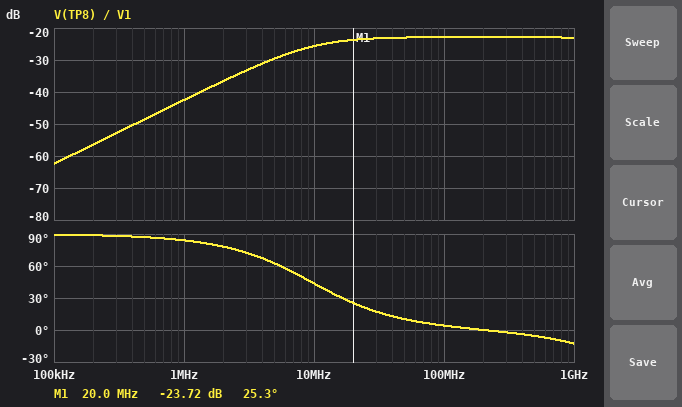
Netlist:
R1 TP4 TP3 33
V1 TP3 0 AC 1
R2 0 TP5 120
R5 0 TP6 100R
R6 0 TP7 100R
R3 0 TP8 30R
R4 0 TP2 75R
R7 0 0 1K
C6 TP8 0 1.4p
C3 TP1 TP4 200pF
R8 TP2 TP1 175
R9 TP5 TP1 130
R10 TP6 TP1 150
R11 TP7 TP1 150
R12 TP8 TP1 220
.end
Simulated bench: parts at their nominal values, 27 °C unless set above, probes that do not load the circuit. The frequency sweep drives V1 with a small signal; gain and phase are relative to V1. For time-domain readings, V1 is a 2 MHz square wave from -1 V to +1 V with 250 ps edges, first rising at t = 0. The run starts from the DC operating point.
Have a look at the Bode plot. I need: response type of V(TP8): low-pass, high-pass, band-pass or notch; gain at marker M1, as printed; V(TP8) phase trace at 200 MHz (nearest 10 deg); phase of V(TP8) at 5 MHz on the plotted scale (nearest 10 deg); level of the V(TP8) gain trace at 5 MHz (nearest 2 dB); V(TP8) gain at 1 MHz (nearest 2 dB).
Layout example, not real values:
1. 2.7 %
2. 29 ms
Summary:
1. high-pass
2. -23.72 dB
3. 0 deg
4. 60 deg
5. -30 dB
6. -42 dB
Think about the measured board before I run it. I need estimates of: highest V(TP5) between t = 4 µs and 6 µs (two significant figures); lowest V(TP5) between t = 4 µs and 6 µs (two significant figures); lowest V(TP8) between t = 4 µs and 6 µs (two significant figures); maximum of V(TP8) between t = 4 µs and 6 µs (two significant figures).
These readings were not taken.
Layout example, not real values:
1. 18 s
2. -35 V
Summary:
1. 570 mV
2. -570 mV
3. -140 mV
4. 140 mV
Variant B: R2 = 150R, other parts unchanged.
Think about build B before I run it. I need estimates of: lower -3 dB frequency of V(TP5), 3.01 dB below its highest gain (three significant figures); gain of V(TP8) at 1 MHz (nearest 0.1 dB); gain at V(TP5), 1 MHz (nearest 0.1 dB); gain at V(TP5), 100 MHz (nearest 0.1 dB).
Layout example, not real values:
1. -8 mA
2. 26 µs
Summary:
1. 9.46 MHz
2. -42.3 dB
3. -29.3 dB
4. -9.8 dB
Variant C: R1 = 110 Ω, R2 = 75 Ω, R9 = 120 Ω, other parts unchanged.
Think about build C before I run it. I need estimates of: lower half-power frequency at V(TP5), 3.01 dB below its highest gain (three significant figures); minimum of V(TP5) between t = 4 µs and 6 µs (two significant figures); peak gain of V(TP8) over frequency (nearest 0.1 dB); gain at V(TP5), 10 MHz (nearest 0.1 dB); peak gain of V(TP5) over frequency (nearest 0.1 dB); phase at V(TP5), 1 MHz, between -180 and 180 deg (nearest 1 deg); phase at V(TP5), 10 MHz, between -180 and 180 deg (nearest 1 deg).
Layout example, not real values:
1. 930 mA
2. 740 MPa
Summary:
1. 5.06 MHz
2. -230 mV
3. -28.9 dB
4. -19.7 dB
5. -18.7 dB
6. 79 deg
7. 27 deg
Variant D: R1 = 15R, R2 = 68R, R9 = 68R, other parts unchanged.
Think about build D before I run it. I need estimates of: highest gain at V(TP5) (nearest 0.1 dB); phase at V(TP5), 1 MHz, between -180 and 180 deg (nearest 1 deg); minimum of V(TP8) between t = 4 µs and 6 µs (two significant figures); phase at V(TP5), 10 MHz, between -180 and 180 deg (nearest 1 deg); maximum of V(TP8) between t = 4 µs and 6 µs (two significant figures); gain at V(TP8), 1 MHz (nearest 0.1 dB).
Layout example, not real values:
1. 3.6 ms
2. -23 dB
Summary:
1. -8.6 dB
2. 86 deg
3. -170 mV
4. 54 deg
5. 170 mV
6. -43.8 dB
